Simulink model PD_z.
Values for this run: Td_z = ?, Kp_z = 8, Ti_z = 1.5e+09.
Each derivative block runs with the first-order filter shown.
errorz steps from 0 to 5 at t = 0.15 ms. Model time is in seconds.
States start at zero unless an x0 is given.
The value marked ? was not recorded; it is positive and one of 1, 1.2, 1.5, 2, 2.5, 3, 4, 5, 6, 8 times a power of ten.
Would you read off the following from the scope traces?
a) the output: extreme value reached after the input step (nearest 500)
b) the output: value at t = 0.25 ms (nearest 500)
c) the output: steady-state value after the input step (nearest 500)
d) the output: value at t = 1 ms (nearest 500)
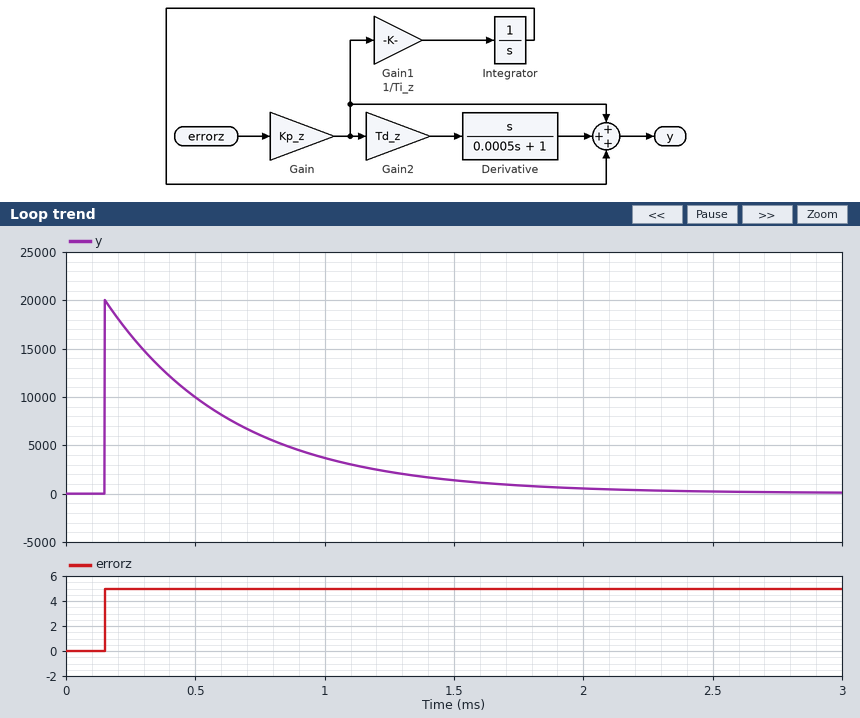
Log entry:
20000
16500
0
3500
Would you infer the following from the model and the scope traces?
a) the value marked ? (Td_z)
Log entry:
0.25
